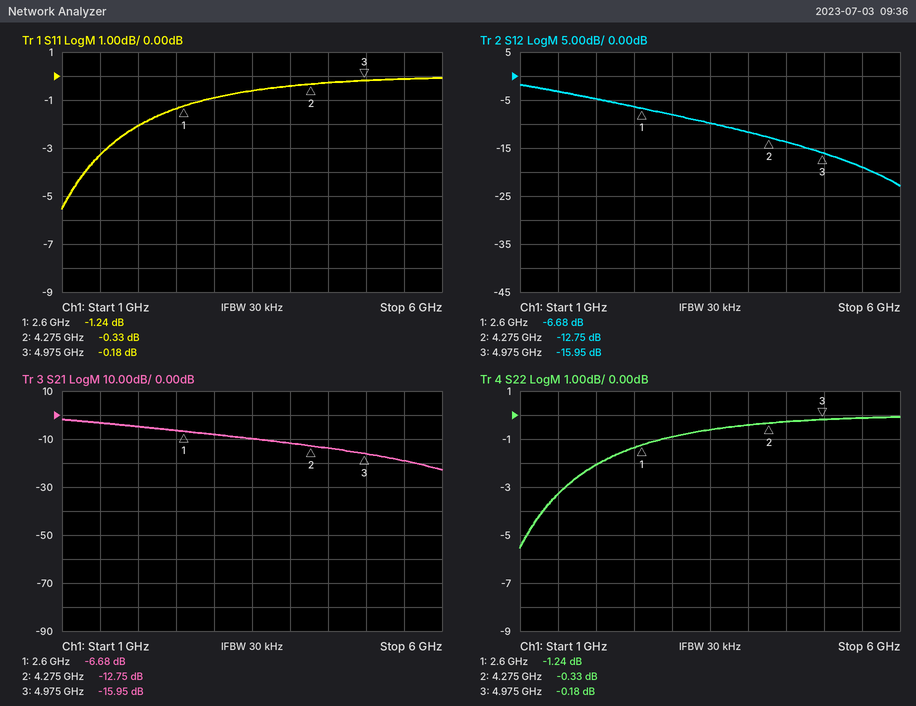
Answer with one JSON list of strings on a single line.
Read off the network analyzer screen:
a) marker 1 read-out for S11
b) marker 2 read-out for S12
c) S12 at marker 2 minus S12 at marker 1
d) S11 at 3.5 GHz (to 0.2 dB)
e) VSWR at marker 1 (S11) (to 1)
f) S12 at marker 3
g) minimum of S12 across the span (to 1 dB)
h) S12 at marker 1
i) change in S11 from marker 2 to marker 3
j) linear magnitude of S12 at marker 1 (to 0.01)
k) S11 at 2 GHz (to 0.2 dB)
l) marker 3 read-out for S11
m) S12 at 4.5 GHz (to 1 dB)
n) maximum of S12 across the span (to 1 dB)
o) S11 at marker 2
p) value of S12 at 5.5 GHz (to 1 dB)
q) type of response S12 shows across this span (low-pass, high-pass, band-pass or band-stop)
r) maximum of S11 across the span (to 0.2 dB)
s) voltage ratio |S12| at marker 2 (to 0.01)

["-1.24 dB", "-12.75 dB", "-6.07 dB", "-0.6 dB", "14", "-15.95 dB", "-23 dB", "-6.68 dB", "0.15 dB", "0.46", "-2.0 dB", "-0.18 dB", "-14 dB", "-2 dB", "-0.33 dB", "-19 dB", "low-pass", "0.0 dB", "0.23"]
